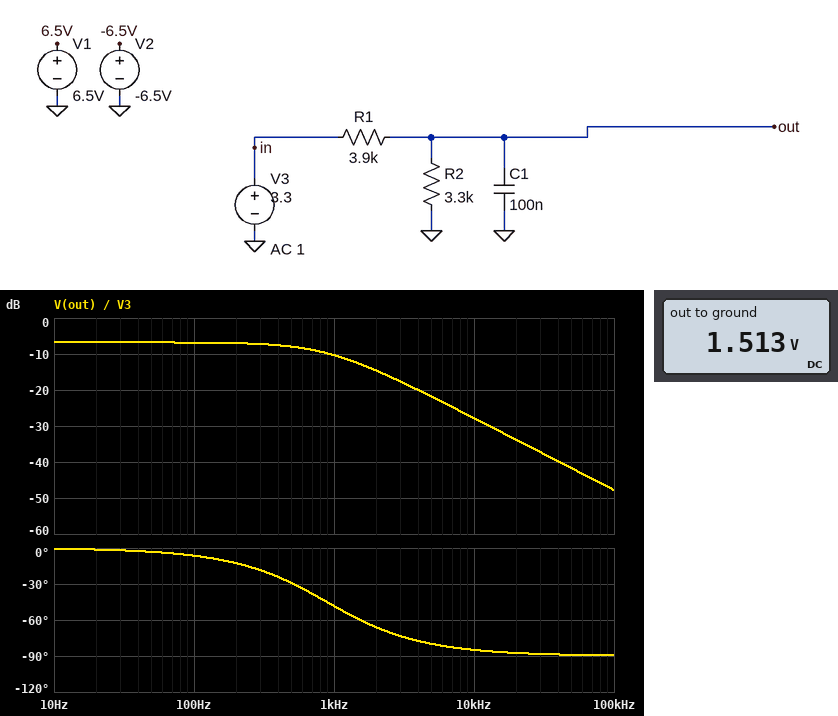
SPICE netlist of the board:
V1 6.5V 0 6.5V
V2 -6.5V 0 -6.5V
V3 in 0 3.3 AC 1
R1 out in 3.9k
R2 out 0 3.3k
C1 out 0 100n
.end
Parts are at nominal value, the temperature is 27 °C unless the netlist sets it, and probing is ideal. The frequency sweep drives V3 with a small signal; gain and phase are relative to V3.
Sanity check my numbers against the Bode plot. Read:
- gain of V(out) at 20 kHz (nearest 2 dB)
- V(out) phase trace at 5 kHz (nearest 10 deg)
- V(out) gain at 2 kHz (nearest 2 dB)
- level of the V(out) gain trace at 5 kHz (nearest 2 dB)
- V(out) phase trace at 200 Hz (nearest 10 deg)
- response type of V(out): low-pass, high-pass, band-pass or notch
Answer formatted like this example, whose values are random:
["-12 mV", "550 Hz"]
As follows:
["-34 dB", "-80 deg", "-14 dB", "-22 dB", "-10 deg", "low-pass"]
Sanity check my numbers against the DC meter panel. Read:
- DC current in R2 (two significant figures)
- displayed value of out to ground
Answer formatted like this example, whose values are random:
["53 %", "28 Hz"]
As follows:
["460 µA", "1.513 V"]
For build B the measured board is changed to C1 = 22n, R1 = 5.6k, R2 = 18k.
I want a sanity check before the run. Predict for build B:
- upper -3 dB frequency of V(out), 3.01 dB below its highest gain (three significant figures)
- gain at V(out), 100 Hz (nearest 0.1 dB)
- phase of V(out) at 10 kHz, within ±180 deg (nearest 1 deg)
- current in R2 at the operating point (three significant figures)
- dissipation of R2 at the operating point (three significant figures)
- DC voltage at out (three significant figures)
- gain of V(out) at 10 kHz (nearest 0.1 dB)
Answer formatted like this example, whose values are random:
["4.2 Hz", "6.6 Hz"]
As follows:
["1.69 kHz", "-2.4 dB", "-80 deg", "140 µA", "352 µW", "2.52 V", "-17.9 dB"]
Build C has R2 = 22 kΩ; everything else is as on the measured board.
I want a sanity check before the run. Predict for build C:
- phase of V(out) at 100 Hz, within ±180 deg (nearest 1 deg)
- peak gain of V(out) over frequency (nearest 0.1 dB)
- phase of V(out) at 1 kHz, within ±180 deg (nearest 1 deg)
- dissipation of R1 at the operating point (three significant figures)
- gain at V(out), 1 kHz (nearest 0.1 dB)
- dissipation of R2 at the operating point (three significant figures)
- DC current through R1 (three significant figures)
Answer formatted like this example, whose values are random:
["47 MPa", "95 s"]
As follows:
["-12 deg", "-1.4 dB", "-64 deg", "63.3 µW", "-8.7 dB", "357 µW", "127 µA"]
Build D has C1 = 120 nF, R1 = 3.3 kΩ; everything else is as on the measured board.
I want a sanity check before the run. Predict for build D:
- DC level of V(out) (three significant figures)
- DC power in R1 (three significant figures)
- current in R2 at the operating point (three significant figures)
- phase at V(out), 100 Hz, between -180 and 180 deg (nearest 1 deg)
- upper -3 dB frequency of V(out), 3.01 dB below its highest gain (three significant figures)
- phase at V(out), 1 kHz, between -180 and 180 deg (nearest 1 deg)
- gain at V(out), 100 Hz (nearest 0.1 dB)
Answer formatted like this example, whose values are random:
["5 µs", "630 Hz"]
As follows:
["1.65 V", "825 µW", "500 µA", "-7 deg", "804 Hz", "-51 deg", "-6.1 dB"]
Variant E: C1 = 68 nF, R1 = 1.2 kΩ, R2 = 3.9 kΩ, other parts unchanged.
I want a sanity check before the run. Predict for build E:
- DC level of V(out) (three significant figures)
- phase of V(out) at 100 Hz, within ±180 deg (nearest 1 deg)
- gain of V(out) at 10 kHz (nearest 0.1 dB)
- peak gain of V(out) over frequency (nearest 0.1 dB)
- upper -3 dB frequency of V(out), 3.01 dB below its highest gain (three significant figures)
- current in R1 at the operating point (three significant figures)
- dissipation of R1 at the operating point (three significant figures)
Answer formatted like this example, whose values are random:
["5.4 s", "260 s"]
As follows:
["2.52 V", "-2 deg", "-14.5 dB", "-2.3 dB", "2.55 kHz", "647 µA", "502 µW"]
